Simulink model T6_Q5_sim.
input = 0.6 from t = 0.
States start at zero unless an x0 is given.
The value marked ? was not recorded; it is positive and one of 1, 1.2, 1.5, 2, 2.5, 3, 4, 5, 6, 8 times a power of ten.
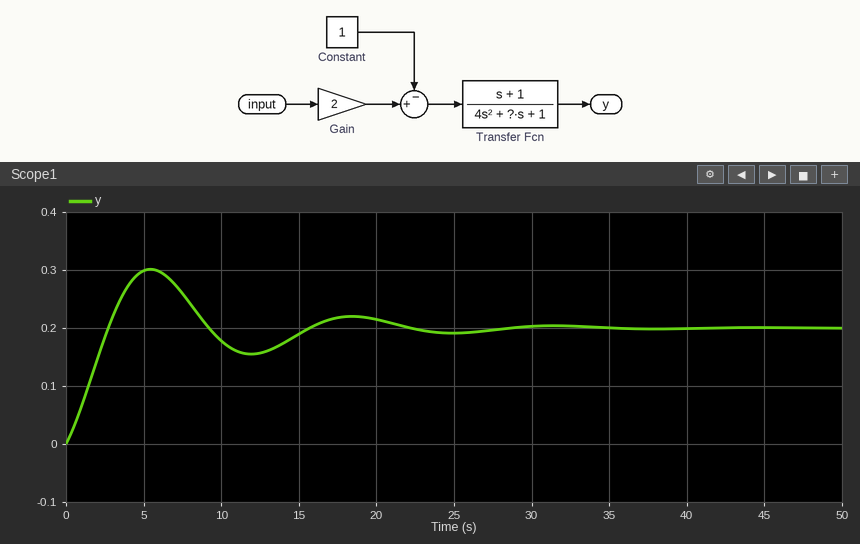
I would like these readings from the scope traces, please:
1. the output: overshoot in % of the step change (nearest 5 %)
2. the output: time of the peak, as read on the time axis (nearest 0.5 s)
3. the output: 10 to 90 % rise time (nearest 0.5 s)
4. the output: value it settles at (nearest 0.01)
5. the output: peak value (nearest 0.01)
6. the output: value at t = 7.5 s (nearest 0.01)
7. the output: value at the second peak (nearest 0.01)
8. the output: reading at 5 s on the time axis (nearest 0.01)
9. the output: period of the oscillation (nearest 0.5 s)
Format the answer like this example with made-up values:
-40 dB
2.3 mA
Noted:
50 %
5.5 s
2.0 s
0.20
0.30
0.26
0.22
0.30
13.0 s
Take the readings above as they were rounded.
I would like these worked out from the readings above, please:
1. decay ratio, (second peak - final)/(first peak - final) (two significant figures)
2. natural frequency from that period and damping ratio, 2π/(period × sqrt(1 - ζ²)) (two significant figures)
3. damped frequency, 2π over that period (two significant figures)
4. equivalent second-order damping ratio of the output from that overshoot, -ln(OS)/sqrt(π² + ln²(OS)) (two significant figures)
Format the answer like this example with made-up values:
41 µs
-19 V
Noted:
0.20
0.50 rad/s
0.48 rad/s
0.22
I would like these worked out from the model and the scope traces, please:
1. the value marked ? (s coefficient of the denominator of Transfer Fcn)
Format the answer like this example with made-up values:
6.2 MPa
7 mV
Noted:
1
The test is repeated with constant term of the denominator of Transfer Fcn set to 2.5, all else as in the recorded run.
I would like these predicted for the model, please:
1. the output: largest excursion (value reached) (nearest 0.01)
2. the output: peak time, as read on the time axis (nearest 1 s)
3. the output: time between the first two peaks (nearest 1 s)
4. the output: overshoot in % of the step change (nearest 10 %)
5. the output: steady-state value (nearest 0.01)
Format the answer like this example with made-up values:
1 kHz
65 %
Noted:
0.14
3 s
8 s
80 %
0.08
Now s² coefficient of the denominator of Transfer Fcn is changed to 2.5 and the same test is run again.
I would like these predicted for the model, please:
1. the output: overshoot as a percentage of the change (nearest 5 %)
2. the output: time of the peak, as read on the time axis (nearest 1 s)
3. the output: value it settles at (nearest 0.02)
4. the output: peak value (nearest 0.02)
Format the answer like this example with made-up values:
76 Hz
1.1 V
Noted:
45 %
4 s
0.20
0.28
